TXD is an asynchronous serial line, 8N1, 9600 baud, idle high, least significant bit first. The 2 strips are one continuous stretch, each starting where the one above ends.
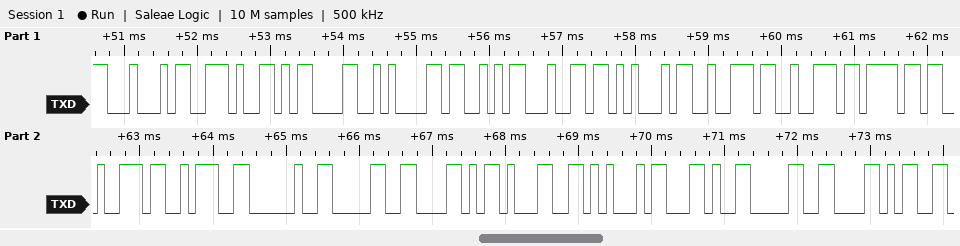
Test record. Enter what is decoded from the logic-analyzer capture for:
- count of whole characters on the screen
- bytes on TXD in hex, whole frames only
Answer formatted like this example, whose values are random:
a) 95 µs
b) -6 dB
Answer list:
a) 20
b) 44 2E 0D 0A 53 64 45 72 72 6F 72 3A 20 30 58 31 45 2C 30 58
